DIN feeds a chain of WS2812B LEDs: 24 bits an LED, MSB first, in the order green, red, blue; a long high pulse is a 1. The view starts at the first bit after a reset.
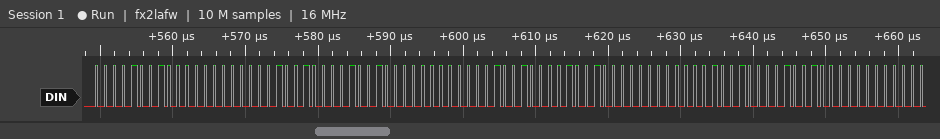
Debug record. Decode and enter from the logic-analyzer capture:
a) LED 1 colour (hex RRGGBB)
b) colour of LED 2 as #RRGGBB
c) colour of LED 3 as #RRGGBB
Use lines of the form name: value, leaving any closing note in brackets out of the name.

LED 1 colour: #000909
colour of LED 2 as #RRGGBB: #000909
colour of LED 3 as #RRGGBB: #000909
